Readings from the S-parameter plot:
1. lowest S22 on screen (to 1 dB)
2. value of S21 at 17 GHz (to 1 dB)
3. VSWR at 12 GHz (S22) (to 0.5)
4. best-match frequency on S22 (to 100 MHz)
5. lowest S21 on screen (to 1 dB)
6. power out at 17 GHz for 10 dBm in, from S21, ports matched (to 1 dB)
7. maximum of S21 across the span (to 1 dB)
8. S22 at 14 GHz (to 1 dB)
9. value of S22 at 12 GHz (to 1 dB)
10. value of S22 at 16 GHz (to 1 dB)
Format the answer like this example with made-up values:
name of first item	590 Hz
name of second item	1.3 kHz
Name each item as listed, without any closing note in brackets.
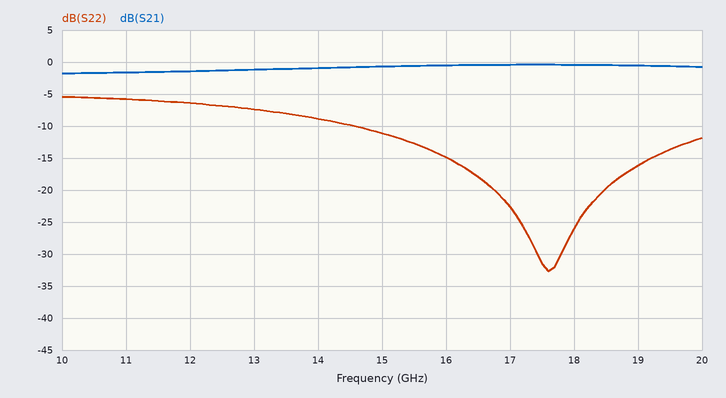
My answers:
lowest S22 on screen	-33 dB
value of S21 at 17 GHz	0 dB
VSWR at 12 GHz (S22)	3.0
best-match frequency on S22	17.6 GHz
lowest S21 on screen	-2 dB
power out at 17 GHz for 10 dBm in, from S21, ports matched	10 dBm
maximum of S21 across the span	0 dB
S22 at 14 GHz	-9 dB
value of S22 at 12 GHz	-6 dB
value of S22 at 16 GHz	-15 dB
